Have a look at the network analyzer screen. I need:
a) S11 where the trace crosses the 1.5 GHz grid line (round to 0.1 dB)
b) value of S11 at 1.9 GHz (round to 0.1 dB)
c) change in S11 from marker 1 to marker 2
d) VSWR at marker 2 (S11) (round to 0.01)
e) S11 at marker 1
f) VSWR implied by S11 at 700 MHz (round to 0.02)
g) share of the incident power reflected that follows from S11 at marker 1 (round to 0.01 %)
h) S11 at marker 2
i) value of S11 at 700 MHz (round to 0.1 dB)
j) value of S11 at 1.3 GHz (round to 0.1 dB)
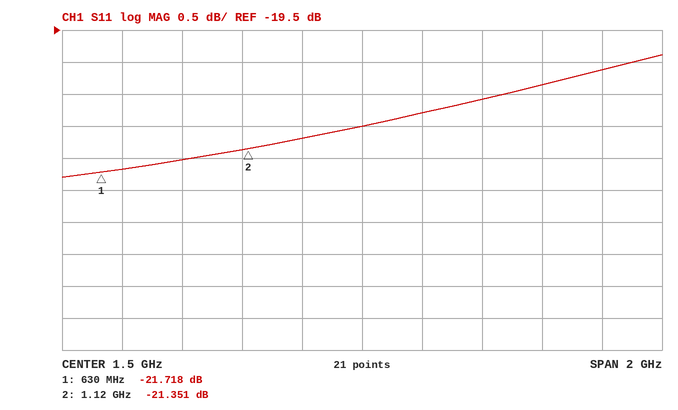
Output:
-21.0 dB
-20.6 dB
0.367 dB
1.19
-21.718 dB
1.18
0.67 %
-21.351 dB
-21.7 dB
-21.2 dB
